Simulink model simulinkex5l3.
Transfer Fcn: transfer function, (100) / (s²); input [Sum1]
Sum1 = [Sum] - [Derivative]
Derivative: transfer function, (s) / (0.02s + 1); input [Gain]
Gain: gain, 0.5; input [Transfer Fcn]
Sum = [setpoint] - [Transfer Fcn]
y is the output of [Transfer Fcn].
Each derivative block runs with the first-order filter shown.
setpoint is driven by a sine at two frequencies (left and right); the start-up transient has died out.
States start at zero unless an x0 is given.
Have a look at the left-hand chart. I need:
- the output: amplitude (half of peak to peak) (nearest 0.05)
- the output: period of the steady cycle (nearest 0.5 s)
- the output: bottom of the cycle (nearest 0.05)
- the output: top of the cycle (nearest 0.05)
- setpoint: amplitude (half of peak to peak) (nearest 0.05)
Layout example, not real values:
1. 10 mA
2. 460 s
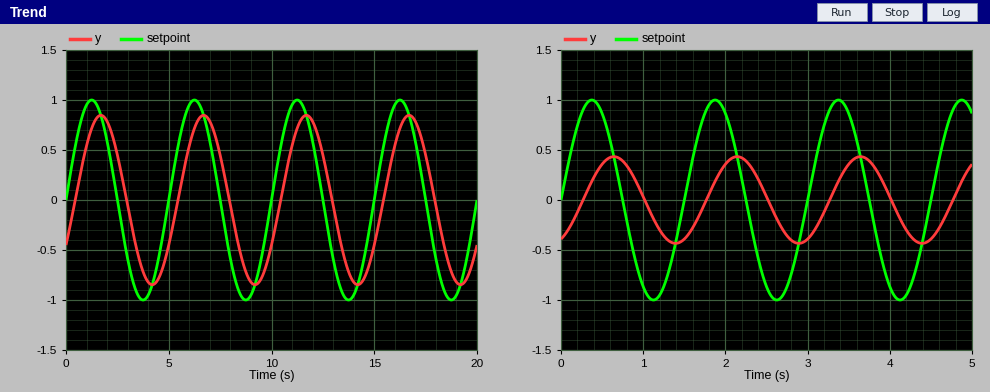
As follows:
1. 0.85
2. 5.0 s
3. -0.85
4. 0.85
5. 1.00
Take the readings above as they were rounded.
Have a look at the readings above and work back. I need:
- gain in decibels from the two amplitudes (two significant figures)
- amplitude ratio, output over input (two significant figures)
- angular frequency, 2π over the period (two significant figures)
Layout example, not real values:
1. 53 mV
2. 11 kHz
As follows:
1. -1.4 dB
2. 0.85
3. 1.3 rad/s
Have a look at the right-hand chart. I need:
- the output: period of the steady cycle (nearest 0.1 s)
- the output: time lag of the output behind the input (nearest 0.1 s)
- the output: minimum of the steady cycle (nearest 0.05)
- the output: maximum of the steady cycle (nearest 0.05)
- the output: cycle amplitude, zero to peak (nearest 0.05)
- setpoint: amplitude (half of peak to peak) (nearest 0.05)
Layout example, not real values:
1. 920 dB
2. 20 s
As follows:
1. 1.5 s
2. 0.3 s
3. -0.45
4. 0.45
5. 0.45
6. 1.00
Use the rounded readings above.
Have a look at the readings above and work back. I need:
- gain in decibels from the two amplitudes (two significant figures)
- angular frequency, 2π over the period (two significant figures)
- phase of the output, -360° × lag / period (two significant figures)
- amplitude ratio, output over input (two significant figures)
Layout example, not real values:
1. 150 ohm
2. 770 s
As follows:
1. -6.9 dB
2. 4.2 rad/s
3. -72°
4. 0.45
